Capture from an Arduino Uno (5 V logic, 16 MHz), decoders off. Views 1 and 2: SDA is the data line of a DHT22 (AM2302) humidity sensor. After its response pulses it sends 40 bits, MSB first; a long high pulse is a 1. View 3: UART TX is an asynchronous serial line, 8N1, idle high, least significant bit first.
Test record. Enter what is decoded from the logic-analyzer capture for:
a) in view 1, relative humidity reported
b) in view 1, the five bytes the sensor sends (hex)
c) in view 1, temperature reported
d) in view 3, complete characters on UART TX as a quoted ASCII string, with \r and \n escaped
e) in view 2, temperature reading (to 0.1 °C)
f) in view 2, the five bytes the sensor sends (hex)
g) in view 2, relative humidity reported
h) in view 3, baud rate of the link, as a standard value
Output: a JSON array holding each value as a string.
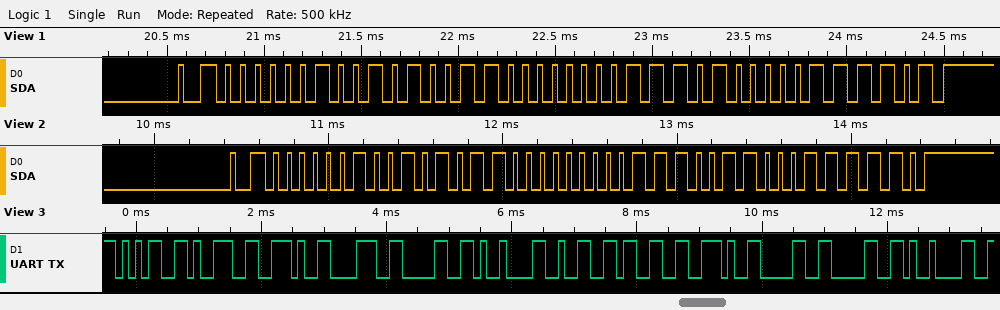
["59.5 %", "02 53 00 E8 3D", "23.2 °C", "\"59.80\\t23.00\\t\"", "23.0 °C", "02 56 00 E6 3E", "59.8 %", "9600 baud"]
